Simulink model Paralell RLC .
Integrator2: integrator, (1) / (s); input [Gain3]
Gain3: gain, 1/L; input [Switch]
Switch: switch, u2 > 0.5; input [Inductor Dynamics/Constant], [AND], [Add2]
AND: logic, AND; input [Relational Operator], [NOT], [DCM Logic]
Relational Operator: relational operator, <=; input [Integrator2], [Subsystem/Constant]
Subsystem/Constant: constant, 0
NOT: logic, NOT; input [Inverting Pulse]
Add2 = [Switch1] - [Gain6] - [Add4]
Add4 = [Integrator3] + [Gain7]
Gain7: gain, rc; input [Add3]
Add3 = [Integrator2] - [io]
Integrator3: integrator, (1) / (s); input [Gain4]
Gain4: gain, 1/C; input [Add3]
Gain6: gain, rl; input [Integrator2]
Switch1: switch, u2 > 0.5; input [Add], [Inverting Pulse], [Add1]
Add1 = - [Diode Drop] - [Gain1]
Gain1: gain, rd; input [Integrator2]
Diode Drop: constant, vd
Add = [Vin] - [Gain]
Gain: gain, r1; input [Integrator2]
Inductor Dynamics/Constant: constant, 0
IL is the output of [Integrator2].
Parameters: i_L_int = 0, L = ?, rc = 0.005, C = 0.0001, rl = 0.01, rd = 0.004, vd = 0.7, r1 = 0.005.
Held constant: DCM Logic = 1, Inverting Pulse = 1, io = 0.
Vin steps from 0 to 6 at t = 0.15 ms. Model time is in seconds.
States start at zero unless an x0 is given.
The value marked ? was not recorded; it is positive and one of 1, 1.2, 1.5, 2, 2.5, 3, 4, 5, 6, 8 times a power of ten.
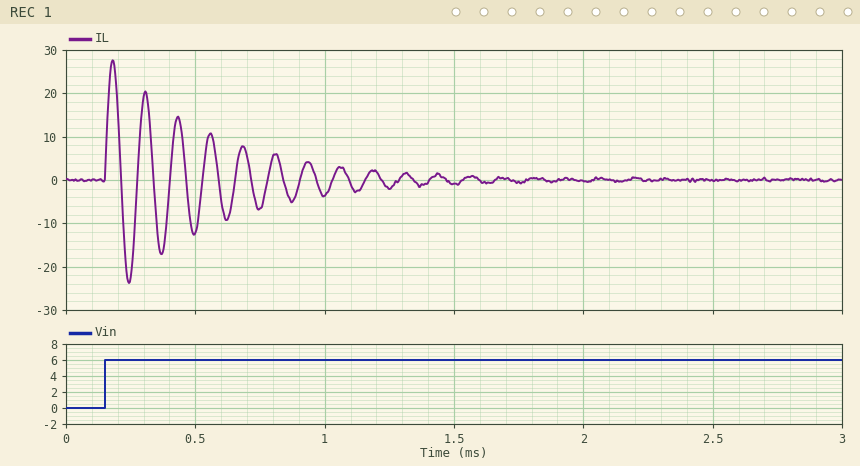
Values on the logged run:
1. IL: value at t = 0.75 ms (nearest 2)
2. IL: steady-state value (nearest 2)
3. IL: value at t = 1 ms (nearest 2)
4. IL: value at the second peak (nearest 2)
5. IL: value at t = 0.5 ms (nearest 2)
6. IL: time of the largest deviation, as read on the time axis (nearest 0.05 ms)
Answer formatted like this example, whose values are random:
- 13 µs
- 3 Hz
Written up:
- -6
- 0
- -4
- 20
- -12
- 0.20 ms
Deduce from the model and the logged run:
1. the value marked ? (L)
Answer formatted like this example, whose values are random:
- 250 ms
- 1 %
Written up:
- 4e-06
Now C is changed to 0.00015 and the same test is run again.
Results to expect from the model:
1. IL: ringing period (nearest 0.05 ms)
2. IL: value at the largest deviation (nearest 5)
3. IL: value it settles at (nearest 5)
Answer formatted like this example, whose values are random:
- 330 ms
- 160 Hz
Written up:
- 0.15 ms
- 35
- 0
